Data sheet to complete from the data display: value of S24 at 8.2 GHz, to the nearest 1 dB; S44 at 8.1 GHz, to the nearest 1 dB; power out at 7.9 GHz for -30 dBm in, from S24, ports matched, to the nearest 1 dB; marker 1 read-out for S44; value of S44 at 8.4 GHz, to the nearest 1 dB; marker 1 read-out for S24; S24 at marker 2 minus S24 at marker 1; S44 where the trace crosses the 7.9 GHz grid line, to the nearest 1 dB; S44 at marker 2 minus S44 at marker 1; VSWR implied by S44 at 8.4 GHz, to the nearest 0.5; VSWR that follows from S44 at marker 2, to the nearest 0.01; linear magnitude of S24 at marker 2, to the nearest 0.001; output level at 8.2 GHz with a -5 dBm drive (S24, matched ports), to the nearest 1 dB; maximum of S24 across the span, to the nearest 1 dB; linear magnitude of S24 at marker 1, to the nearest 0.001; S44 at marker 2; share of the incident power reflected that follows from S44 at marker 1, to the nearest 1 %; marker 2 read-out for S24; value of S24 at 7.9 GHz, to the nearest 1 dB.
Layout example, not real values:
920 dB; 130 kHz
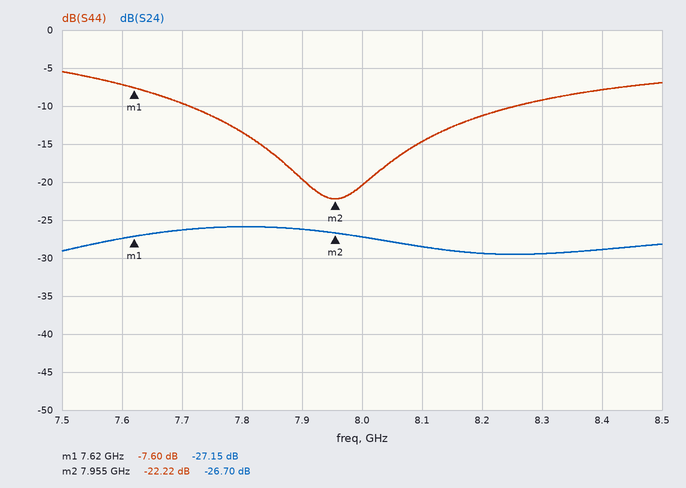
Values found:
-29 dB; -15 dB; -56 dBm; -7.60 dB; -8 dB; -27.15 dB; 0.45 dB; -20 dB; -14.62 dB; 2.5; 1.17; 0.046; -34 dBm; -26 dB; 0.044; -22.22 dB; 17 %; -26.70 dB; -26 dB
